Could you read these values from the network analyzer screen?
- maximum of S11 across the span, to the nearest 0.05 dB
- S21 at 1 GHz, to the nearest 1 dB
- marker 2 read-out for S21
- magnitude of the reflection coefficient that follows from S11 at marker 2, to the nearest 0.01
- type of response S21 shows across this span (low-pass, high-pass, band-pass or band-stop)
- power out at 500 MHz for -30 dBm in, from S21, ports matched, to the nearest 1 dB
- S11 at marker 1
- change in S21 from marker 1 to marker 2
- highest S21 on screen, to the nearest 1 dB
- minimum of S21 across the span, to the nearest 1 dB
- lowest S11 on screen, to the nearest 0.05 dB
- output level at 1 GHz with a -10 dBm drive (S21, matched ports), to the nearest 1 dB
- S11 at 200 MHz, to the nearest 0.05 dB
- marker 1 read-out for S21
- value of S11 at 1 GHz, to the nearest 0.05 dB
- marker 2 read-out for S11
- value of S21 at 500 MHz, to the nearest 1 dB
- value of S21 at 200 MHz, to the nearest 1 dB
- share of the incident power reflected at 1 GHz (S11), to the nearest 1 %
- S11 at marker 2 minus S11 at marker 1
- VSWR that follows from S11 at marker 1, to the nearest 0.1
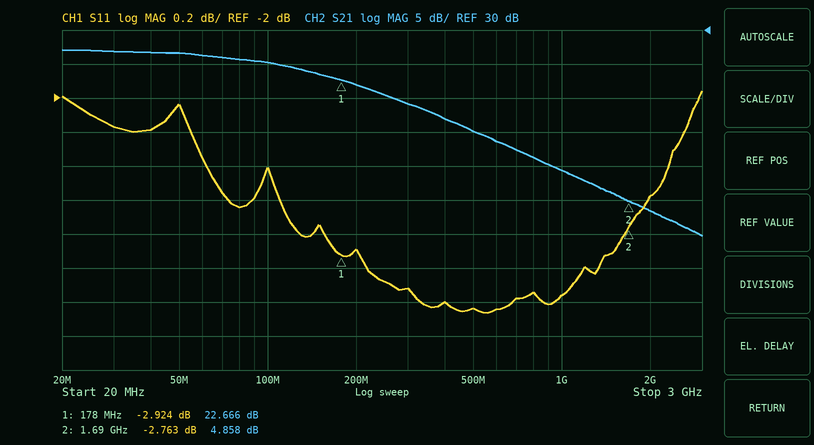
-1.95 dB
9 dB
4.858 dB
0.73
low-pass
-15 dBm
-2.924 dB
-17.808 dB
27 dB
0 dB
-3.25 dB
-1 dBm
-2.90 dB
22.666 dB
-3.15 dB
-2.763 dB
15 dB
22 dB
48 %
0.161 dB
6.0
